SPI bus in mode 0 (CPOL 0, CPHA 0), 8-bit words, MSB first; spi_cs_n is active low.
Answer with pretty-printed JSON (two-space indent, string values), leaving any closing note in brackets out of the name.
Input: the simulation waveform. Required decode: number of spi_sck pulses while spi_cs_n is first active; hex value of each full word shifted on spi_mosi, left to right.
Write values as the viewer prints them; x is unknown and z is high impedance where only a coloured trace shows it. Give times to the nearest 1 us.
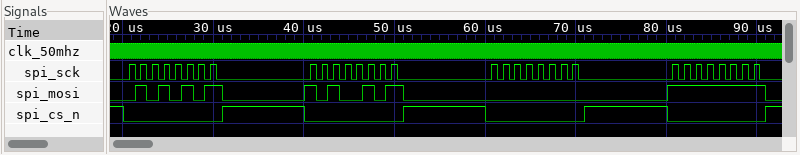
{
  "number of spi_sck pulses while spi_cs_n is first active": "8",
  "hex value of each full word shifted on spi_mosi, left to right": "55, A5, 00, FF"
}
